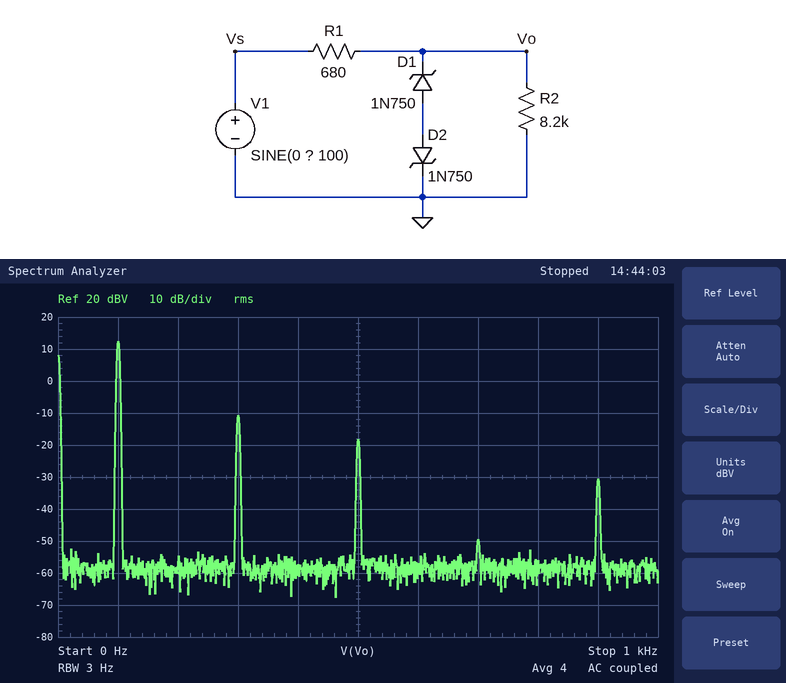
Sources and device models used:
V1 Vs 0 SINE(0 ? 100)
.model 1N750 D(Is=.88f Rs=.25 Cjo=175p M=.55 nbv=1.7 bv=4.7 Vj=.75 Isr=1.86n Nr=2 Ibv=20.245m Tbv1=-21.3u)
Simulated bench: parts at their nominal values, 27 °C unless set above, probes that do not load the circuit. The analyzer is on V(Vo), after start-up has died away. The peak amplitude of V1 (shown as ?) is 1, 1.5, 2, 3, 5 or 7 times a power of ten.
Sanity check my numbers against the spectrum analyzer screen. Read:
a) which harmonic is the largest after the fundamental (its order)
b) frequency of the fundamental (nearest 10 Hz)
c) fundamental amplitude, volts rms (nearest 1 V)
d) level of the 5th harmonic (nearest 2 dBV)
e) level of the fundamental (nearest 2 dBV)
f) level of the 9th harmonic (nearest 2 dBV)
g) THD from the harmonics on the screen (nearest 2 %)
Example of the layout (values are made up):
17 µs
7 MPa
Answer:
3
100 Hz
4 V
-18 dBV
12 dBV
-30 dBV
8 %
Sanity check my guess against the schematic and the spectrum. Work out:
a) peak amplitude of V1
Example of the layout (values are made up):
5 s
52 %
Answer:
7 V
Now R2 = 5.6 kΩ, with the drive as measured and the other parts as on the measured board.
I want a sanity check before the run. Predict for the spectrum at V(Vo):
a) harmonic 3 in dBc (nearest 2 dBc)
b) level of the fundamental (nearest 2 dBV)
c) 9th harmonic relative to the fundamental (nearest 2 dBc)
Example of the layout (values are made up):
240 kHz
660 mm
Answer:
-24 dBc
12 dBV
-46 dBc
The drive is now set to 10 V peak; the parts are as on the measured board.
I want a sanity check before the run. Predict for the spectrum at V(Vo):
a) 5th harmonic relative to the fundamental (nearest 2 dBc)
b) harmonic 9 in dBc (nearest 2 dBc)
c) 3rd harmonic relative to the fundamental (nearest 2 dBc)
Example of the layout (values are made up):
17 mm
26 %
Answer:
-38 dBc
-38 dBc
-14 dBc
